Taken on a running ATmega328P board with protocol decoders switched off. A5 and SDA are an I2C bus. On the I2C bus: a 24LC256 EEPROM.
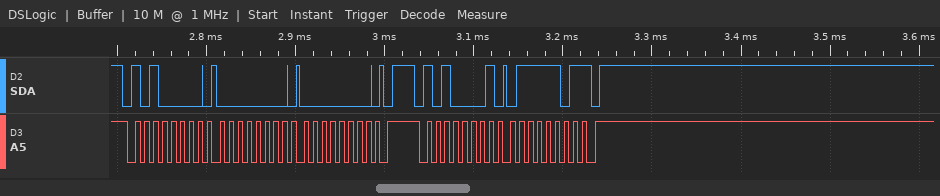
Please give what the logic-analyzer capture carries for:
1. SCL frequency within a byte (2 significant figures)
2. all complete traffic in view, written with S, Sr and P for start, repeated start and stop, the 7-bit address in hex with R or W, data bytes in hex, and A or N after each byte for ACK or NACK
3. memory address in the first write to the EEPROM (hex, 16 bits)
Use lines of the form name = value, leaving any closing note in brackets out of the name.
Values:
SCL frequency within a byte = 100 kHz
all complete traffic in view, written with S, Sr and P for start, repeated start and stop, the 7-bit address in hex with R or W, data bytes in hex, and A or N after each byte for ACK or NACK = S 50W A 00 A 00 A P S 50R A 7D N P
memory address in the first write to the EEPROM = 0x0000
